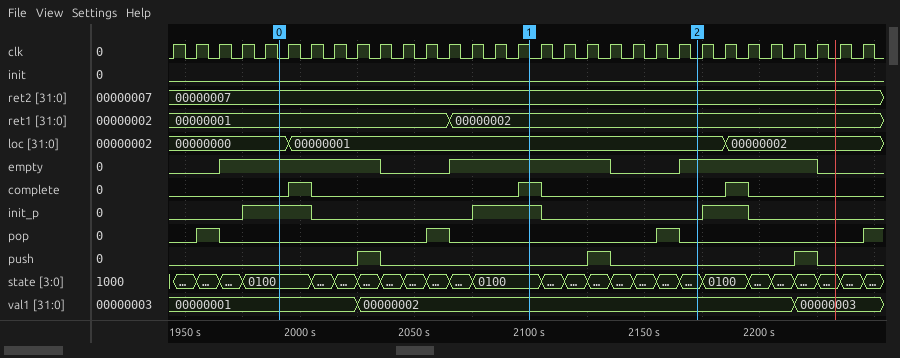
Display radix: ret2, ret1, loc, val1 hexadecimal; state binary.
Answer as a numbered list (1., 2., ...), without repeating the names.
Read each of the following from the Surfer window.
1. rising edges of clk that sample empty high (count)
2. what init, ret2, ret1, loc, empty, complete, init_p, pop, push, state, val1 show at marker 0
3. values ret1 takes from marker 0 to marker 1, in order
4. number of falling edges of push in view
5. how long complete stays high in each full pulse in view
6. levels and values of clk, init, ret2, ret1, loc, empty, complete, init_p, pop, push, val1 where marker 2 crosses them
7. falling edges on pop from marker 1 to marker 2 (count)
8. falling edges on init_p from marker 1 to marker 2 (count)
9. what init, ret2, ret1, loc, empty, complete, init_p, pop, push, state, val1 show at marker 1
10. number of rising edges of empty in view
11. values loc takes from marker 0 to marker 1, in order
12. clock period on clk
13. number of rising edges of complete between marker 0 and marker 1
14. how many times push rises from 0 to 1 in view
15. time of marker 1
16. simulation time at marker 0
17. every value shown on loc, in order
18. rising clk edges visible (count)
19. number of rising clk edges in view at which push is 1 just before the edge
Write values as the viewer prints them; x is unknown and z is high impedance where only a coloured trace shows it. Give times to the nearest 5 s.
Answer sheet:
1. 20
2. init=0, ret2=00000007, ret1=00000001, loc=00000000, empty=1, complete=0, init_p=1, pop=0, push=0, state=0100, val1=00000001
3. 00000001, 00000002
4. 3
5. 10 s, 10 s, 10 s
6. clk=0, init=0, ret2=00000007, ret1=00000002, loc=00000001, empty=1, complete=0, init_p=0, pop=0, push=0, val1=00000002
7. 1
8. 1
9. init=0, ret2=00000007, ret1=00000002, loc=00000001, empty=1, complete=1, init_p=1, pop=0, push=0, state=0100, val1=00000002
10. 3
11. 00000000, 00000001
12. 10 s
13. 2
14. 3
15. 2100 s
16. 1990 s
17. 00000000, 00000001, 00000002
18. 31
19. 3
